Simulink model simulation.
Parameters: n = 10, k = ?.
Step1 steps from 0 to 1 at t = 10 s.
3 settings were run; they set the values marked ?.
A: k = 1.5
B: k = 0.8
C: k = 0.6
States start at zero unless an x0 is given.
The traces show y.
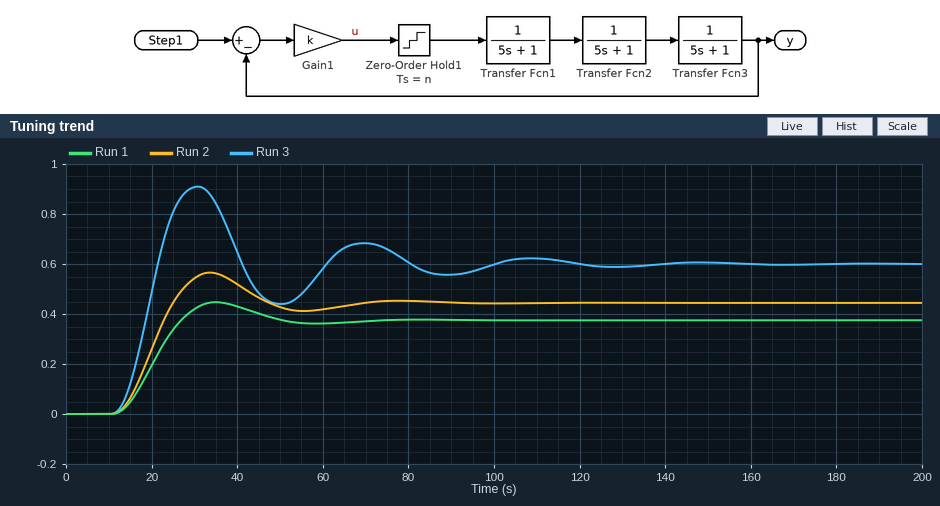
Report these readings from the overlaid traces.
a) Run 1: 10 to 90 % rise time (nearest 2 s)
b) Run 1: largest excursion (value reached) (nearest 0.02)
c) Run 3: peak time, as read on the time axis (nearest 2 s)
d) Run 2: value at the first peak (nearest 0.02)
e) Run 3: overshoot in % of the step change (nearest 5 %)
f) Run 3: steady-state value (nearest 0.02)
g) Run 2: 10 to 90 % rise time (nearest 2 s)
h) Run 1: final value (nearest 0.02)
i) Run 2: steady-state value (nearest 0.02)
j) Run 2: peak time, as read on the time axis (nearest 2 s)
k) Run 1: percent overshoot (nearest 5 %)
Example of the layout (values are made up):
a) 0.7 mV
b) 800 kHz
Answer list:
a) 10 s
b) 0.44
c) 30 s
d) 0.56
e) 50 %
f) 0.60
g) 10 s
h) 0.38
i) 0.44
j) 34 s
k) 20 %
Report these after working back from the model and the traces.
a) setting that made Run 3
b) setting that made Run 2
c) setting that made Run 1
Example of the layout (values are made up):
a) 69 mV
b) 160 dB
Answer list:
a) A
b) B
c) C
